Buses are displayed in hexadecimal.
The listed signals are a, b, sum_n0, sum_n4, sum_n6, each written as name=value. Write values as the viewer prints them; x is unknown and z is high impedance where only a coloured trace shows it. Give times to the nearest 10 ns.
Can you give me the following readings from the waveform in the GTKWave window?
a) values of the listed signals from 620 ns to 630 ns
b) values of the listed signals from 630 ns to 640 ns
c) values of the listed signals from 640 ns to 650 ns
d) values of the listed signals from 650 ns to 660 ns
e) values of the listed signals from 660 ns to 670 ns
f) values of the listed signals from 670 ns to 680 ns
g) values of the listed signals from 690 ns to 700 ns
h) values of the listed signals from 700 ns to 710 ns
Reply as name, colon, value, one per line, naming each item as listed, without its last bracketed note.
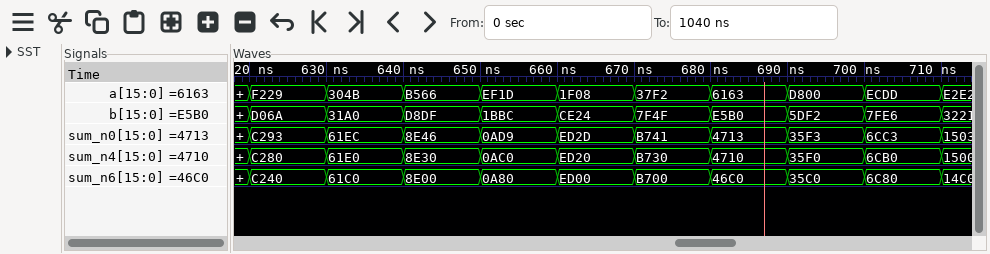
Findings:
values of the listed signals from 620 ns to 630 ns: a=F229, b=D06A, sum_n0=C293, sum_n4=C280, sum_n6=C240
values of the listed signals from 630 ns to 640 ns: a=304B, b=31A0, sum_n0=61EC, sum_n4=61E0, sum_n6=61C0
values of the listed signals from 640 ns to 650 ns: a=B566, b=D8DF, sum_n0=8E46, sum_n4=8E30, sum_n6=8E00
values of the listed signals from 650 ns to 660 ns: a=EF1D, b=1BBC, sum_n0=0AD9, sum_n4=0AC0, sum_n6=0A80
values of the listed signals from 660 ns to 670 ns: a=1F08, b=CE24, sum_n0=ED2D, sum_n4=ED20, sum_n6=ED00
values of the listed signals from 670 ns to 680 ns: a=37F2, b=7F4F, sum_n0=B741, sum_n4=B730, sum_n6=B700
values of the listed signals from 690 ns to 700 ns: a=D800, b=5DF2, sum_n0=35F3, sum_n4=35F0, sum_n6=35C0
values of the listed signals from 700 ns to 710 ns: a=ECDD, b=7FE6, sum_n0=6CC3, sum_n4=6CB0, sum_n6=6C80
